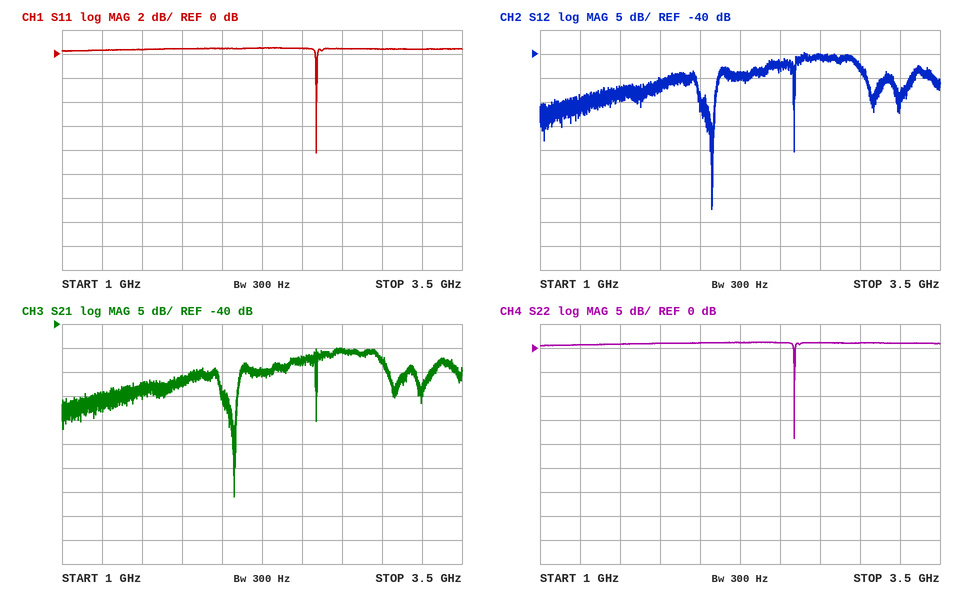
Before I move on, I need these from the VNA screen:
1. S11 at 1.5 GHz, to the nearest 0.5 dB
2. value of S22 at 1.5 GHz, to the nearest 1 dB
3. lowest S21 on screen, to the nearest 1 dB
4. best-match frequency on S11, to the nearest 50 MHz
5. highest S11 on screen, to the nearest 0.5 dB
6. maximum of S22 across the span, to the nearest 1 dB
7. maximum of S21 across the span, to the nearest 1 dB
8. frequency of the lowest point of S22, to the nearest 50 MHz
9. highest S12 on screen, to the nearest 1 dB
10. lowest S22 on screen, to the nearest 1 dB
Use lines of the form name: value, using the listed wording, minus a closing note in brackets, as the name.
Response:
S11 at 1.5 GHz, to the nearest 0.5 dB: 0.5 dB
value of S22 at 1.5 GHz, to the nearest 1 dB: 1 dB
lowest S21 on screen, to the nearest 1 dB: -76 dB
best-match frequency on S11, to the nearest 50 MHz: 2.60 GHz
highest S11 on screen, to the nearest 0.5 dB: 0.5 dB
maximum of S22 across the span, to the nearest 1 dB: 1 dB
maximum of S21 across the span, to the nearest 1 dB: -45 dB
frequency of the lowest point of S22, to the nearest 50 MHz: 2.60 GHz
highest S12 on screen, to the nearest 1 dB: -40 dB
lowest S22 on screen, to the nearest 1 dB: -19 dB
